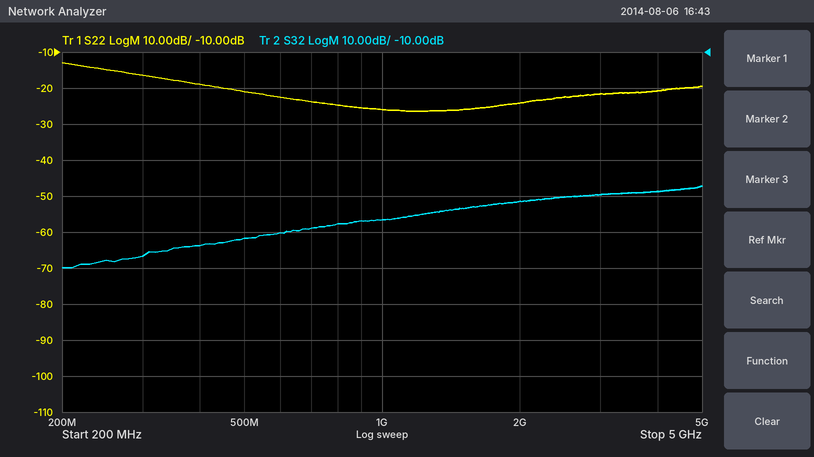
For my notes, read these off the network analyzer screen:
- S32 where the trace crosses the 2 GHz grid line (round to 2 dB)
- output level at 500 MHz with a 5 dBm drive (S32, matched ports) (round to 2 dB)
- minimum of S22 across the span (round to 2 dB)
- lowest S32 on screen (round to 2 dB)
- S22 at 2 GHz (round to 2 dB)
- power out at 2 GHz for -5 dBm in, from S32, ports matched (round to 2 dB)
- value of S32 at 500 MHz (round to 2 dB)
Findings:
-52 dB
-56 dBm
-26 dB
-70 dB
-24 dB
-56 dBm
-62 dB
